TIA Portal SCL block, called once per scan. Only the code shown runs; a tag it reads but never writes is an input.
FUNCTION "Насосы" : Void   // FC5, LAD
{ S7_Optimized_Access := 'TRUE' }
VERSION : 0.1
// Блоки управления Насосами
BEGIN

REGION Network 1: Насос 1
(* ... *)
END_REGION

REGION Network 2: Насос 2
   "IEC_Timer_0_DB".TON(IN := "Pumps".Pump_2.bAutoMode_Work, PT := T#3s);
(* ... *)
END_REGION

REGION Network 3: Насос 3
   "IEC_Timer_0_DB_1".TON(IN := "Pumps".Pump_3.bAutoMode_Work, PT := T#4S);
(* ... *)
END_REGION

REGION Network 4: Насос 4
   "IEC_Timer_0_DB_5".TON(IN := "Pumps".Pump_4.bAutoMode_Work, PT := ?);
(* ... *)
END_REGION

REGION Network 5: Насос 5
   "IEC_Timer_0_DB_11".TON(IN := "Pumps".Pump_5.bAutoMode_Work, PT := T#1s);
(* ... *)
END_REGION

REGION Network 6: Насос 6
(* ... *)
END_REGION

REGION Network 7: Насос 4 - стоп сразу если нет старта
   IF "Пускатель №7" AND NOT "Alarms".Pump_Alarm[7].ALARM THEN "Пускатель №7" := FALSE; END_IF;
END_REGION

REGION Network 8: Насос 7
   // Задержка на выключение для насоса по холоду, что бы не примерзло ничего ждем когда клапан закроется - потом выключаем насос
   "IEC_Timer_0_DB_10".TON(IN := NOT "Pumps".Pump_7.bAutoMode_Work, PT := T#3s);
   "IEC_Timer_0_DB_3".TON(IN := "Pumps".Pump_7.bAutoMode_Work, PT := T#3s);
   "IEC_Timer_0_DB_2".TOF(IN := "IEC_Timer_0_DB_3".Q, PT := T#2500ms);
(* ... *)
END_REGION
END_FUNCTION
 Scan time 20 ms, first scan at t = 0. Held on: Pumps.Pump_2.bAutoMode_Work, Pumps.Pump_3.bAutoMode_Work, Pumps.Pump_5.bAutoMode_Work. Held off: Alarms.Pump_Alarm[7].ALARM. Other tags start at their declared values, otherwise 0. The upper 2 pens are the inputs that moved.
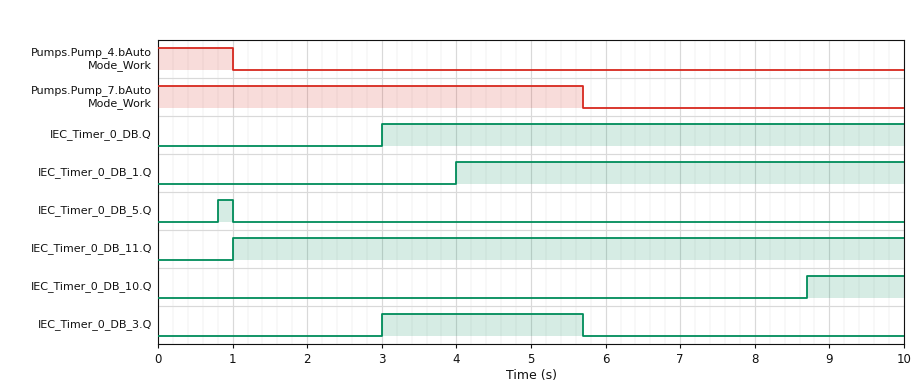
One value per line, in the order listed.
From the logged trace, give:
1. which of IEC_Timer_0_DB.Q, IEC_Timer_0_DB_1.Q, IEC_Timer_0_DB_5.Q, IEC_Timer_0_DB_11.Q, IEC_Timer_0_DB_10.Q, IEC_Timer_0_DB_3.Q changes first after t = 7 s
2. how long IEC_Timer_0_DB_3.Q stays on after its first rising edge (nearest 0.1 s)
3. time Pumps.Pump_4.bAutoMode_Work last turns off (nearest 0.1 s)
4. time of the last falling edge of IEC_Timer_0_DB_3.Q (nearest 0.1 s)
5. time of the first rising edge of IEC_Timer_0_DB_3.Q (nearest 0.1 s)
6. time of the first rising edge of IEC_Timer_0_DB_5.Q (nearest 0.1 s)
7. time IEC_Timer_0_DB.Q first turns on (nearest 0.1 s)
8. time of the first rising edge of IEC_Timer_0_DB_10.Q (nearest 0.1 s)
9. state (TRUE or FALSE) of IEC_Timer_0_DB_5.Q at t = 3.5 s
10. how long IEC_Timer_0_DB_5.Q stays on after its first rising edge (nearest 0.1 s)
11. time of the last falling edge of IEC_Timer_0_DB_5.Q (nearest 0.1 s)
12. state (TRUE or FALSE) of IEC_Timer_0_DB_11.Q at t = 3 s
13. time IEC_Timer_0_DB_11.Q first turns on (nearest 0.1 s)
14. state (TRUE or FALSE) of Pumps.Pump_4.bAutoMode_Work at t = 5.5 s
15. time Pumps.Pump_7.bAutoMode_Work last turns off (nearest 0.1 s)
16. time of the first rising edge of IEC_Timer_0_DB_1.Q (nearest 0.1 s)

IEC_Timer_0_DB_10.Q
2.7 s
1.0 s
5.7 s
3.0 s
0.8 s
3.0 s
8.7 s
FALSE
0.2 s
1.0 s
TRUE
1.0 s
FALSE
5.7 s
4.0 s
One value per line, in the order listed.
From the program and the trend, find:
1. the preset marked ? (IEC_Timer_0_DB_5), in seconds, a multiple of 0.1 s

0.8 s
